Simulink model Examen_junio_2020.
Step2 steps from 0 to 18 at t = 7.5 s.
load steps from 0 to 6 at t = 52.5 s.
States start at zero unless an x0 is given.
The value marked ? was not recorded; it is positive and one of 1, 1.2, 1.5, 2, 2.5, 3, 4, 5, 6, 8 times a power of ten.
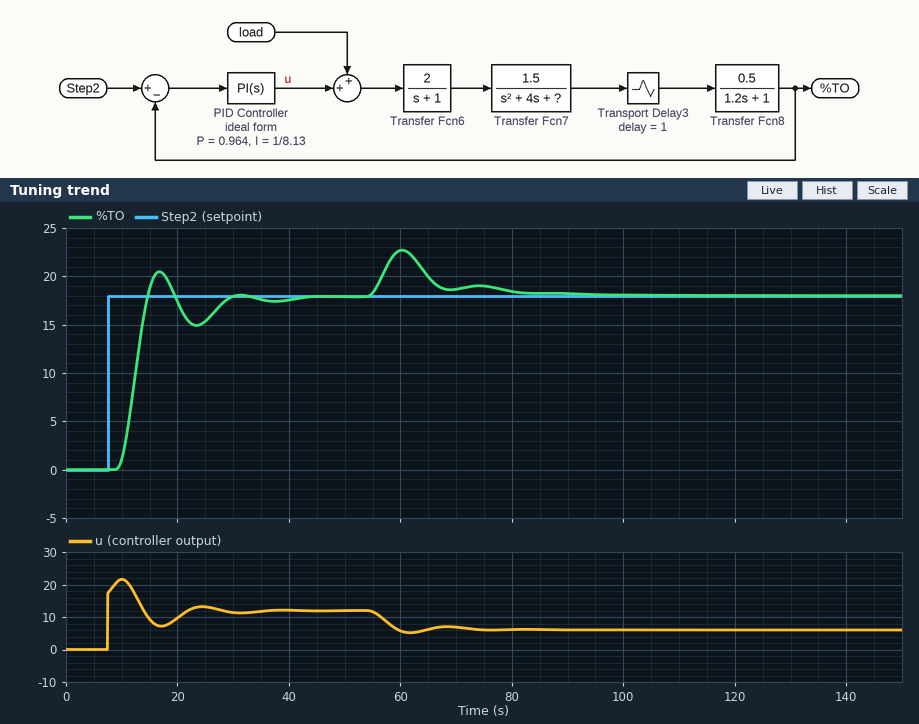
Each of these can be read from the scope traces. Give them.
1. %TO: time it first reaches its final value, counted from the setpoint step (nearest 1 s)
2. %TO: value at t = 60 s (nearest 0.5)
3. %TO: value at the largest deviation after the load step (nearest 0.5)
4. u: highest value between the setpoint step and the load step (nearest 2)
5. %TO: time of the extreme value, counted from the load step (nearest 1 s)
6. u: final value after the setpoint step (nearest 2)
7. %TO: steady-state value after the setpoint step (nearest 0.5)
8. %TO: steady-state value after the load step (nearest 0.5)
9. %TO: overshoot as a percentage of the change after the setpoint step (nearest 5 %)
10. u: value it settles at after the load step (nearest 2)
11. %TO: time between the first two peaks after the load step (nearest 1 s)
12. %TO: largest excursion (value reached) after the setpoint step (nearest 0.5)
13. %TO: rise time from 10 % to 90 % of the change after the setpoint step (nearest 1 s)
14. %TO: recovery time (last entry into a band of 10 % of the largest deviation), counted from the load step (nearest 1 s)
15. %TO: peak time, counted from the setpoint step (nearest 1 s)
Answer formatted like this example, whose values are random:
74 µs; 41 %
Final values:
7 s; 22.5; 22.5; 22; 8 s; 12; 18.0; 18.0; 15 %; 6; 14 s; 20.5; 4 s; 27 s; 9 s
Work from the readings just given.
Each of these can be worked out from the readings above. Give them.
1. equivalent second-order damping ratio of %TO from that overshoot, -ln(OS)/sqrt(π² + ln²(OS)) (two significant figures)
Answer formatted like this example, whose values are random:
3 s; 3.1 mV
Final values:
0.52
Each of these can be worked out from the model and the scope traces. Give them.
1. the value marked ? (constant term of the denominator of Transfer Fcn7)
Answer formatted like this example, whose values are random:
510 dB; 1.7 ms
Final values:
1
